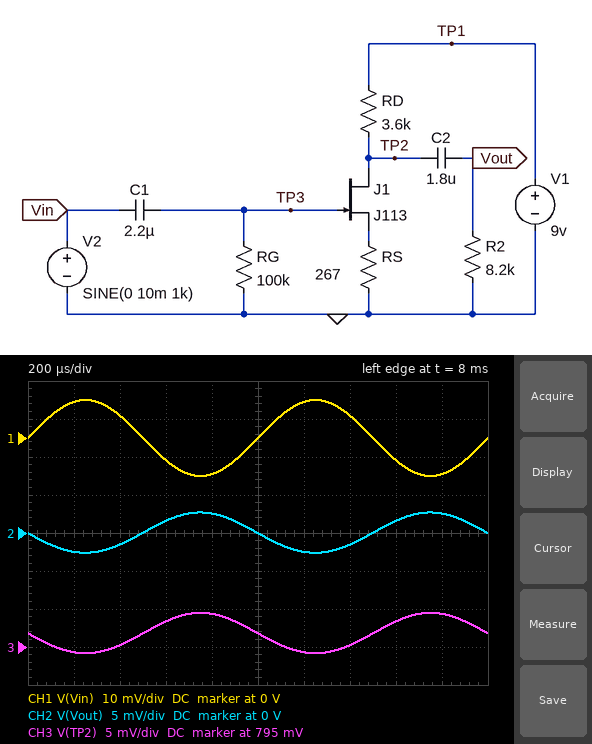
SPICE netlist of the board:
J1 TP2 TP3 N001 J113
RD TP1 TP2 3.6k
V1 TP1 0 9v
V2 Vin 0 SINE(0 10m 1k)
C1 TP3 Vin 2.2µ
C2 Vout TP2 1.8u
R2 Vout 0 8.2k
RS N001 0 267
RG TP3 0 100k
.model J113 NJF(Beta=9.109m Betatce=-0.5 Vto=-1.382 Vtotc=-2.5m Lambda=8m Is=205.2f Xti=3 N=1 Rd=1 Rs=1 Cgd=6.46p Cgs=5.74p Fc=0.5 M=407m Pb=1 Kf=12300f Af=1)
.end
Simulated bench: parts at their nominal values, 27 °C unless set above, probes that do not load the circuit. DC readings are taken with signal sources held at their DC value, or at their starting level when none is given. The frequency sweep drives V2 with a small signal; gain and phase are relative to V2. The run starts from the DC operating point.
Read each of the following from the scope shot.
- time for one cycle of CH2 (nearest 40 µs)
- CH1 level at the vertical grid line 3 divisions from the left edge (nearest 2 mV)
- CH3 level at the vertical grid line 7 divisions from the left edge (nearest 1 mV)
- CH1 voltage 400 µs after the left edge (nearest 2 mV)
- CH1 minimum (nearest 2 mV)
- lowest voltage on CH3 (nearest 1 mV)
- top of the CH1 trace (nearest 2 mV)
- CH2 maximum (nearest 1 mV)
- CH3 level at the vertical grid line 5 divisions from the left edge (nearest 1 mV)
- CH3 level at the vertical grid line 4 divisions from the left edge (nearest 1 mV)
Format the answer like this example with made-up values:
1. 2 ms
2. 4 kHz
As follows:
1. 1.00 ms
2. -6 mV
3. 795 mV
4. 6 mV
5. -10 mV
6. 794 mV
7. 10 mV
8. 3 mV
9. 797 mV
10. 799 mV
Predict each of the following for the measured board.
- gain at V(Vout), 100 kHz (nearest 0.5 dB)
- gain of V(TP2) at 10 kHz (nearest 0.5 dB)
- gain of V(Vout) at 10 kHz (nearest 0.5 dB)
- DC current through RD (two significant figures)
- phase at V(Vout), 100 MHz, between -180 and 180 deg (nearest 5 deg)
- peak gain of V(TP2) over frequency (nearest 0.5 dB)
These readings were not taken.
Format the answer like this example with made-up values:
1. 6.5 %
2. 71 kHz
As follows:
1. -11.5 dB
2. -11.5 dB
3. -11.5 dB
4. 2.3 mA
5. 40 deg
6. 0.5 dB
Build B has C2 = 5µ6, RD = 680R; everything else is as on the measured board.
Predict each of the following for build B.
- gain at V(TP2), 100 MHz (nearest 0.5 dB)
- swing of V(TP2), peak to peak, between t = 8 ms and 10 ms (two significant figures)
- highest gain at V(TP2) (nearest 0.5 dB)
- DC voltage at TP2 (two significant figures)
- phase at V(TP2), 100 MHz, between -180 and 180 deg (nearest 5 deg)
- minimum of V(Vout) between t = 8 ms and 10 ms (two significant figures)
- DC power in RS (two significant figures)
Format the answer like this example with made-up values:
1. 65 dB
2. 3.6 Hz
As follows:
1. 3.5 dB
2. 35 mV
3. 5.0 dB
4. 6.9 V
5. 100 deg
6. -17 mV
7. 2.5 mW
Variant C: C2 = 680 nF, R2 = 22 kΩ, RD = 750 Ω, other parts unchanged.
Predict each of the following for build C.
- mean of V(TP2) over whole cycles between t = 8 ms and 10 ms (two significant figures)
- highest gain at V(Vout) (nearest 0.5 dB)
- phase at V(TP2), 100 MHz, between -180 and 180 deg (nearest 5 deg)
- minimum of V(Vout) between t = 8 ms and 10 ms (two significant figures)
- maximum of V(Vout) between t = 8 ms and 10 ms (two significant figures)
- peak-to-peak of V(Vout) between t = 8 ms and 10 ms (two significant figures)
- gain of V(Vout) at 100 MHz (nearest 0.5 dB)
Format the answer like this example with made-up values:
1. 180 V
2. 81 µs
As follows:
1. 6.7 V
2. 6.0 dB
3. 95 deg
4. -20 mV
5. 20 mV
6. 40 mV
7. 4.5 dB
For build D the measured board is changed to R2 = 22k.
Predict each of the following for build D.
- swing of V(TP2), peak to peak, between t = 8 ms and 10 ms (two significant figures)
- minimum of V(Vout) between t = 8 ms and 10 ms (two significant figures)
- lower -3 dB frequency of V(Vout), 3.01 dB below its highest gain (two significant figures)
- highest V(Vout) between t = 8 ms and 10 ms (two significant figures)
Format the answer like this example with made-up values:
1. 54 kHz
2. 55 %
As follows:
1. 5.5 mV
2. -2.7 mV
3. 51 MHz
4. 2.8 mV
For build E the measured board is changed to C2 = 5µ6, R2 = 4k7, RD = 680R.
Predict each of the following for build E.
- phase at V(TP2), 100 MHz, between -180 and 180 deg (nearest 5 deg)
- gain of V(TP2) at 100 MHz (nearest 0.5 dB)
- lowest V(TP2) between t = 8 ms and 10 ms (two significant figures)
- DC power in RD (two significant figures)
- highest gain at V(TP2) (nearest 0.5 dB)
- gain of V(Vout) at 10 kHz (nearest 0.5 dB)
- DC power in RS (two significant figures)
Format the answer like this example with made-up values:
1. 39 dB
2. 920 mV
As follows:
1. 105 deg
2. 3.5 dB
3. 6.9 V
4. 6.3 mW
5. 5.0 dB
6. 4.5 dB
7. 2.5 mW
